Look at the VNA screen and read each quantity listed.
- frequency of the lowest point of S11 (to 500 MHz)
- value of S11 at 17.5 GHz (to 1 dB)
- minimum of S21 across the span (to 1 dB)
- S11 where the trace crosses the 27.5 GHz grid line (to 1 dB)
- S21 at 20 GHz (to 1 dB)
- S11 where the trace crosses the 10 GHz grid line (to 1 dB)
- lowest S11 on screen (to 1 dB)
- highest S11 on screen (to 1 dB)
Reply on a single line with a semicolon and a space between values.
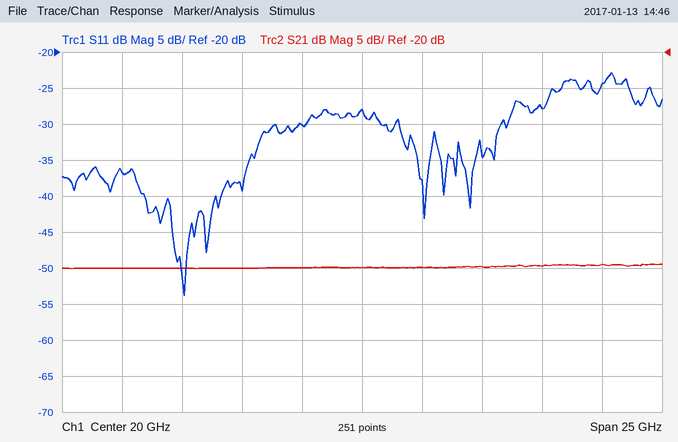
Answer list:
12.5 GHz; -30 dB; -50 dB; -28 dB; -50 dB; -37 dB; -54 dB; -23 dB
